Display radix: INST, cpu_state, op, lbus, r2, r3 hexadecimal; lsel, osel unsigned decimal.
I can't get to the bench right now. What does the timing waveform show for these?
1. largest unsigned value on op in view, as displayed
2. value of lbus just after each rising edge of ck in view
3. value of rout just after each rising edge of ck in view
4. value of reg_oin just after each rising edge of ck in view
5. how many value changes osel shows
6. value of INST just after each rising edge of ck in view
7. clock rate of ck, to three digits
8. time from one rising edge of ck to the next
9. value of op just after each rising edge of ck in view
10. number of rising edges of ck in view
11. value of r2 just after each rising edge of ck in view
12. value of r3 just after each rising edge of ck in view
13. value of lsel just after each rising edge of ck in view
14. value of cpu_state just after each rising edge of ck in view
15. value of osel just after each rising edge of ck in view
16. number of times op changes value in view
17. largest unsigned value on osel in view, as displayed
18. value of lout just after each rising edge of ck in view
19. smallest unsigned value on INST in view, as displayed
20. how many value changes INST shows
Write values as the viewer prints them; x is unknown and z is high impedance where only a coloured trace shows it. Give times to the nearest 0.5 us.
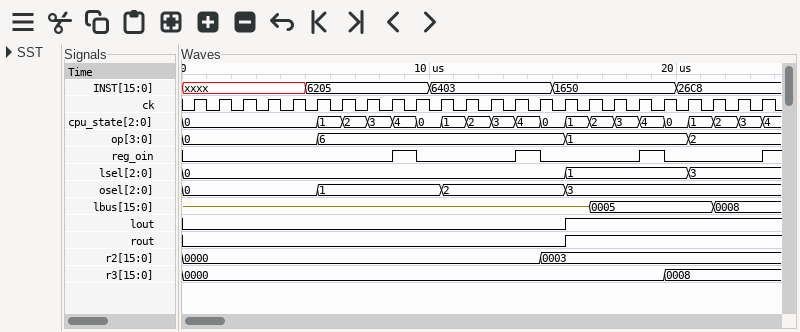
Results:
6
z, z, z, z, z, z, z, z, z, z, z, z, z, z, z, z, 0005, 0005, 0005, 0005, 0005, 0008, 0008, 0008
0 0 0 0 0 0 0 0 0 0 0 0 0 0 0 1 1 1 1 1 1 1 1 1
0 0 0 0 0 0 0 0 1 0 0 0 0 1 0 0 0 0 1 0 0 0 0 1
3
xxxx, xxxx, xxxx, xxxx, xxxx, 6205, 6205, 6205, 6205, 6205, 6403, 6403, 6403, 6403, 6403, 1650, 1650, 1650, 1650, 1650, 26C8, 26C8, 26C8, 26C8
1.00 MHz
1 us
0, 0, 0, 0, 0, 6, 6, 6, 6, 6, 6, 6, 6, 6, 6, 1, 1, 1, 1, 1, 2, 2, 2, 2
24
0000, 0000, 0000, 0000, 0000, 0000, 0000, 0000, 0000, 0000, 0000, 0000, 0000, 0000, 0003, 0003, 0003, 0003, 0003, 0003, 0003, 0003, 0003, 0003
0000, 0000, 0000, 0000, 0000, 0000, 0000, 0000, 0000, 0000, 0000, 0000, 0000, 0000, 0000, 0000, 0000, 0000, 0000, 0008, 0008, 0008, 0008, 0008
0, 0, 0, 0, 0, 0, 0, 0, 0, 0, 0, 0, 0, 0, 0, 1, 1, 1, 1, 1, 3, 3, 3, 3
0, 0, 0, 0, 0, 1, 2, 3, 4, 0, 1, 2, 3, 4, 0, 1, 2, 3, 4, 0, 1, 2, 3, 4
0, 0, 0, 0, 0, 1, 1, 1, 1, 1, 2, 2, 2, 2, 2, 3, 3, 3, 3, 3, 3, 3, 3, 3
3
3
0 0 0 0 0 0 0 0 0 0 0 0 0 0 0 1 1 1 1 1 1 1 1 1
1650
4
